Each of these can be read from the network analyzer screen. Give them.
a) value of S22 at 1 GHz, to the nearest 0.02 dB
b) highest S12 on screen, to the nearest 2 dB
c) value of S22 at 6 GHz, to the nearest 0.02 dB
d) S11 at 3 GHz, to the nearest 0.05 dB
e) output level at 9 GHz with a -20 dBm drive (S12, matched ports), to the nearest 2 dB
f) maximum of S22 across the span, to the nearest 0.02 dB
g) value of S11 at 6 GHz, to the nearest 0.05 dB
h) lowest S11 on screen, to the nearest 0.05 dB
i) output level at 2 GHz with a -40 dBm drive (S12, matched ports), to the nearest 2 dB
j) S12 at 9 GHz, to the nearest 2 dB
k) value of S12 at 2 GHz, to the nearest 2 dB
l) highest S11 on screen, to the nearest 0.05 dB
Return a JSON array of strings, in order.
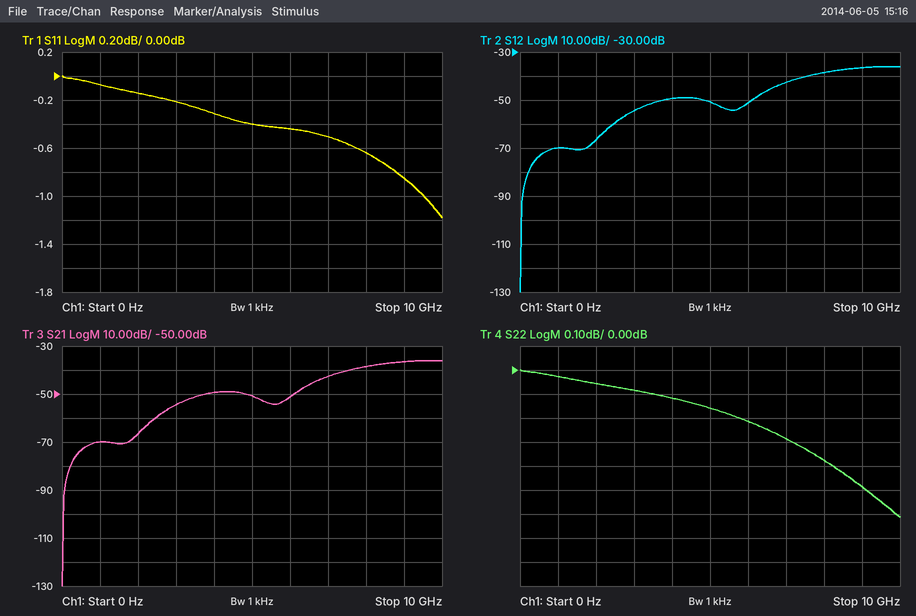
["-0.02 dB", "-36 dB", "-0.22 dB", "-0.20 dB", "-56 dBm", "0.00 dB", "-0.45 dB", "-1.20 dB", "-106 dBm", "-36 dB", "-66 dB", "0.00 dB"]
